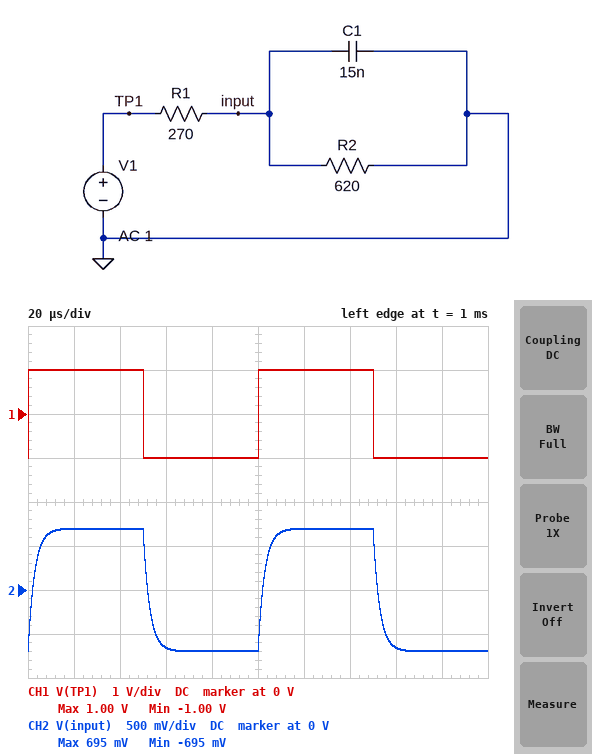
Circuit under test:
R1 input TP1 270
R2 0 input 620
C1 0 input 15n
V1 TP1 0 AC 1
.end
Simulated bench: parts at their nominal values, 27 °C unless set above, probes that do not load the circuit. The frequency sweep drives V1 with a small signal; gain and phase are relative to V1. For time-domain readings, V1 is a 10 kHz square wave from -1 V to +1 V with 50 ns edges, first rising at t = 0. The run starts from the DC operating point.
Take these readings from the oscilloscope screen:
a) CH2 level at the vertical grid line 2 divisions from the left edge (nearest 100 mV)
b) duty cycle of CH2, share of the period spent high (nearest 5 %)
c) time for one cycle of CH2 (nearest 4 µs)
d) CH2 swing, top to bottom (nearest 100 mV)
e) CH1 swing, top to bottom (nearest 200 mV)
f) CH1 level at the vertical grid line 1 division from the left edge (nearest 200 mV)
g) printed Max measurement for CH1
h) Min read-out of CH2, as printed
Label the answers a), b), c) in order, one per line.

a) 700 mV
b) 50 %
c) 100 µs
d) 1.4 V
e) 2.0 V
f) 1.0 V
g) 1.00 V
h) -695 mV
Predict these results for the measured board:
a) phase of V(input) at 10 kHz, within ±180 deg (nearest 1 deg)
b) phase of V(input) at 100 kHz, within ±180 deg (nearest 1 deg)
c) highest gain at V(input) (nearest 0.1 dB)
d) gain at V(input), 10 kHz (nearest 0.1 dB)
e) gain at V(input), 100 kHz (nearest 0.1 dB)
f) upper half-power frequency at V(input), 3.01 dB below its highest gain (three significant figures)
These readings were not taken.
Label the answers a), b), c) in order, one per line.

a) -10 deg
b) -61 deg
c) -3.1 dB
d) -3.3 dB
e) -9.3 dB
f) 56.4 kHz
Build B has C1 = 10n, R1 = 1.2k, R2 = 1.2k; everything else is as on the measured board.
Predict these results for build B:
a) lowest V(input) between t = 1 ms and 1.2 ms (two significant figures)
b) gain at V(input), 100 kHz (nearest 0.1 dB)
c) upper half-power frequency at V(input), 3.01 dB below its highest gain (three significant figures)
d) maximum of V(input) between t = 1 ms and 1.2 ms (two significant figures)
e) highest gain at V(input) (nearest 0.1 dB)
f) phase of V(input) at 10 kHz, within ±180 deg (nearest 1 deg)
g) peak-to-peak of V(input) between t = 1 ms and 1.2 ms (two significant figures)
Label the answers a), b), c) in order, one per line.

a) -500 mV
b) -17.8 dB
c) 26.5 kHz
d) 500 mV
e) -6.0 dB
f) -21 deg
g) 1.0 V
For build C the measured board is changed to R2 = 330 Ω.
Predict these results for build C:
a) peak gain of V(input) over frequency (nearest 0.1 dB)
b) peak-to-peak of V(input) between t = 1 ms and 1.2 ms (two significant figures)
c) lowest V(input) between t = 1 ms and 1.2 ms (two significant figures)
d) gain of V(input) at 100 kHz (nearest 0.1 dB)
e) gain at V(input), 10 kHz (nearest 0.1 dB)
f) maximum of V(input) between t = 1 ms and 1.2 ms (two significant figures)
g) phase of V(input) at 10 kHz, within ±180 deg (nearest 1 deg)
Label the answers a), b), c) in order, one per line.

a) -5.2 dB
b) 1.1 V
c) -550 mV
d) -9.9 dB
e) -5.3 dB
f) 550 mV
g) -8 deg
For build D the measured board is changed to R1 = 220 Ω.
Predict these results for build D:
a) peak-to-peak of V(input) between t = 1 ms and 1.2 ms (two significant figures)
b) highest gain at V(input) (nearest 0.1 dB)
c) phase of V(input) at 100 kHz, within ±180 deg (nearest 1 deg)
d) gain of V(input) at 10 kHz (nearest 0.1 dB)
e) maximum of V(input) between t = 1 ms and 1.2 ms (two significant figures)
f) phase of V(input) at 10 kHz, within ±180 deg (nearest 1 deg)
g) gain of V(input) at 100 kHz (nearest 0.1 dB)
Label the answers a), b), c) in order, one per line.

a) 1.5 V
b) -2.6 dB
c) -57 deg
d) -2.7 dB
e) 740 mV
f) -9 deg
g) -7.9 dB
